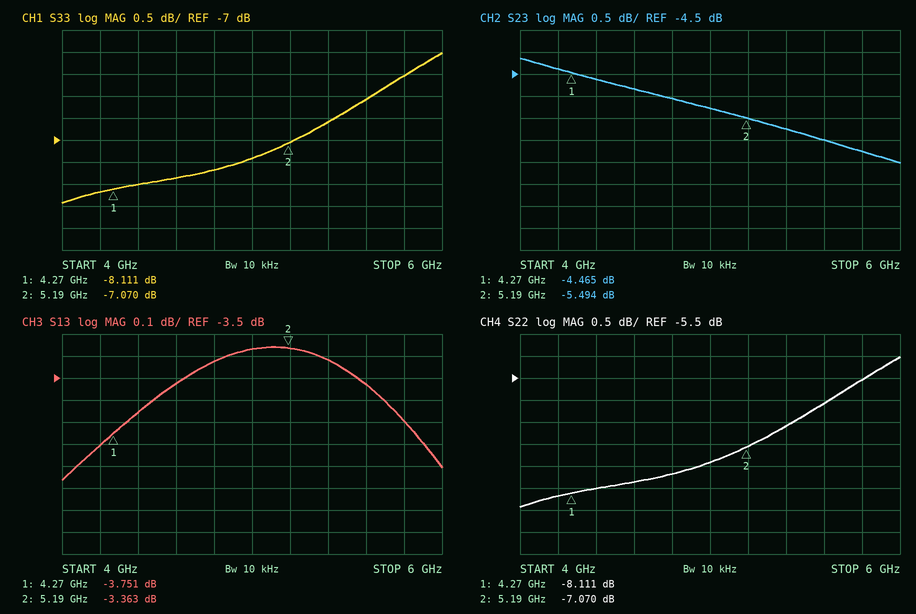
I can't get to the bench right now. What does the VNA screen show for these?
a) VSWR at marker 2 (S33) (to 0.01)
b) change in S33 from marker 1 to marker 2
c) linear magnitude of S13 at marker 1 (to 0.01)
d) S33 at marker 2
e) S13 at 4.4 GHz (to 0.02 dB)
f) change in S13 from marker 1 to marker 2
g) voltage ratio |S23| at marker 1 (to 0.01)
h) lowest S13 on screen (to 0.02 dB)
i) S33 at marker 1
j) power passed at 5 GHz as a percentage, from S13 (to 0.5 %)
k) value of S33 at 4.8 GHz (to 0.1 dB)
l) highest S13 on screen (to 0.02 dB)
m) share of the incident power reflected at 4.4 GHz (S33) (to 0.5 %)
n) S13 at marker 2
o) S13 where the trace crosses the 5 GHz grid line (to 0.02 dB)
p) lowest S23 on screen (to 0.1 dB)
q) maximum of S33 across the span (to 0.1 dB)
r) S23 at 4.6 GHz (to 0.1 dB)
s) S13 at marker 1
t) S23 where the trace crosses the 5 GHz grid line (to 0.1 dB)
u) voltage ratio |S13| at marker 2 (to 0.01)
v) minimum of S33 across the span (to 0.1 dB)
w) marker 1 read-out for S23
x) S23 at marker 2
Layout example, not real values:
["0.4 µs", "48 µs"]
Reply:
["2.59", "1.041 dB", "0.65", "-7.070 dB", "-3.66 dB", "0.388 dB", "0.60", "-3.96 dB", "-8.111 dB", "46.0 %", "-7.7 dB", "-3.36 dB", "16.0 %", "-3.363 dB", "-3.36 dB", "-6.5 dB", "-5.0 dB", "-4.8 dB", "-3.751 dB", "-5.3 dB", "0.68", "-8.4 dB", "-4.465 dB", "-5.494 dB"]
